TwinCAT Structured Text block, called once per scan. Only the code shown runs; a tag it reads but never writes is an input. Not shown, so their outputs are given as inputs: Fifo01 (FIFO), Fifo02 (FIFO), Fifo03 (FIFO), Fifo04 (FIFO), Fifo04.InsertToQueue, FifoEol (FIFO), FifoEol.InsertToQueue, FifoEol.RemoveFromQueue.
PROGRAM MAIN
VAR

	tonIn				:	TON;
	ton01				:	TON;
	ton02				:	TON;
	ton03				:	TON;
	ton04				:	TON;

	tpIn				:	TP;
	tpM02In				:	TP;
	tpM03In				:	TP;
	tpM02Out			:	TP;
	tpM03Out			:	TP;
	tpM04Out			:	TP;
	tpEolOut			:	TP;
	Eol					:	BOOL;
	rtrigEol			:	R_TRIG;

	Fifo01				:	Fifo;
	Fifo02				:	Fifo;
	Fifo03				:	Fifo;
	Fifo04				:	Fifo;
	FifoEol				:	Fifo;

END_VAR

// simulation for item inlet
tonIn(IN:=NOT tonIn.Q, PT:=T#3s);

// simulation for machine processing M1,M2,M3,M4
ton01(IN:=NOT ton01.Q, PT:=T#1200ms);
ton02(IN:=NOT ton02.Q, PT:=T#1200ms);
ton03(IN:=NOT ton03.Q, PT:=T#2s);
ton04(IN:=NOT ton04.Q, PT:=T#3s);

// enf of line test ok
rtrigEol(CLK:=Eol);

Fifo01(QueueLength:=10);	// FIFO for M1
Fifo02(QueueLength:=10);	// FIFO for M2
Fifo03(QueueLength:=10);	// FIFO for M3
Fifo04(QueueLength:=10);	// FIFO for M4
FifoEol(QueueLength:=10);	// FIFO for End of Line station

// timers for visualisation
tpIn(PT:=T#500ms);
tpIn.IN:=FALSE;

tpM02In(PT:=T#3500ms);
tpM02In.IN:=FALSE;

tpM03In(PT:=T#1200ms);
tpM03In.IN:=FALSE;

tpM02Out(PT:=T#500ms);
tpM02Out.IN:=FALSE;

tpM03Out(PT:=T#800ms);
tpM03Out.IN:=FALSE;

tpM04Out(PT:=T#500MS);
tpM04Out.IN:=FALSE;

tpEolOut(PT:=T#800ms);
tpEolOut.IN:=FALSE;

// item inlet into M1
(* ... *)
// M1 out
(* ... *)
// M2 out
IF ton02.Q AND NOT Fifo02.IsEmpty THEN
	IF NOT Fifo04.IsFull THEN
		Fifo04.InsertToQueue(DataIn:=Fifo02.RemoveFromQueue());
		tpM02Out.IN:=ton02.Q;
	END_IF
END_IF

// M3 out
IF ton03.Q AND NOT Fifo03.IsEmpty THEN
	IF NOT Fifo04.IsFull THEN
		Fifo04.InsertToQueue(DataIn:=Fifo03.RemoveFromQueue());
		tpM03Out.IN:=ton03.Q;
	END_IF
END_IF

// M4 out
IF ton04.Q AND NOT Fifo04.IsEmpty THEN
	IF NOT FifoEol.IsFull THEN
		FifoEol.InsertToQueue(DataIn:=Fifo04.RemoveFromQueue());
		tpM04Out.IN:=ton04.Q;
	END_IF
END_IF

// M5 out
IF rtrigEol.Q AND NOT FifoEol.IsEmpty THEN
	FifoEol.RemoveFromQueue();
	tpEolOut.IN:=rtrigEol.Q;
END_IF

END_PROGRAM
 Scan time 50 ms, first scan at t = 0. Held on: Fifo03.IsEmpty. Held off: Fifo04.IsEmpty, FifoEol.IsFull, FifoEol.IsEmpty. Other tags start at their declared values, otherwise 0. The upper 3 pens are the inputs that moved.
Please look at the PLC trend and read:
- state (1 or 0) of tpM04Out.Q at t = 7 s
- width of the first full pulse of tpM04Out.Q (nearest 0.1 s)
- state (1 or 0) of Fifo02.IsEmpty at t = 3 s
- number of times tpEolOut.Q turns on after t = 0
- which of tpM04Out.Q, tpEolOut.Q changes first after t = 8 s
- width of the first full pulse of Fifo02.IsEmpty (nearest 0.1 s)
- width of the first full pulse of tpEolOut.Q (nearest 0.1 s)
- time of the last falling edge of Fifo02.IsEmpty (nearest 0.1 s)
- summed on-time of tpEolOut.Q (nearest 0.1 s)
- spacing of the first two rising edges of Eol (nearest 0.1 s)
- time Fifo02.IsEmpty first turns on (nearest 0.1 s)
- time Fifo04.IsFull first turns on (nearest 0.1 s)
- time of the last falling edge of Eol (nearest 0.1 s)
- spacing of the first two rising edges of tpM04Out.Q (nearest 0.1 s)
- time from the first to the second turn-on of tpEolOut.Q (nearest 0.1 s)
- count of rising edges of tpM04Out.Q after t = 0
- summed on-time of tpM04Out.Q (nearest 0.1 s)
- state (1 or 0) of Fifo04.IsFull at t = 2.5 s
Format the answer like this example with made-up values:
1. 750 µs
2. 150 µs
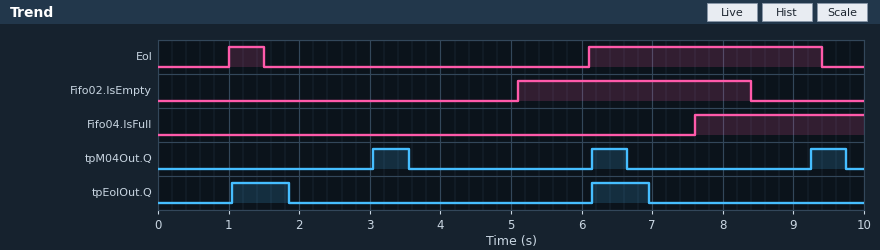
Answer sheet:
1. 0
2. 0.5 s
3. 0
4. 2
5. tpM04Out.Q
6. 3.3 s
7. 0.8 s
8. 8.4 s
9. 1.6 s
10. 5.1 s
11. 5.1 s
12. 7.6 s
13. 9.4 s
14. 3.1 s
15. 5.1 s
16. 3
17. 1.5 s
18. 0
